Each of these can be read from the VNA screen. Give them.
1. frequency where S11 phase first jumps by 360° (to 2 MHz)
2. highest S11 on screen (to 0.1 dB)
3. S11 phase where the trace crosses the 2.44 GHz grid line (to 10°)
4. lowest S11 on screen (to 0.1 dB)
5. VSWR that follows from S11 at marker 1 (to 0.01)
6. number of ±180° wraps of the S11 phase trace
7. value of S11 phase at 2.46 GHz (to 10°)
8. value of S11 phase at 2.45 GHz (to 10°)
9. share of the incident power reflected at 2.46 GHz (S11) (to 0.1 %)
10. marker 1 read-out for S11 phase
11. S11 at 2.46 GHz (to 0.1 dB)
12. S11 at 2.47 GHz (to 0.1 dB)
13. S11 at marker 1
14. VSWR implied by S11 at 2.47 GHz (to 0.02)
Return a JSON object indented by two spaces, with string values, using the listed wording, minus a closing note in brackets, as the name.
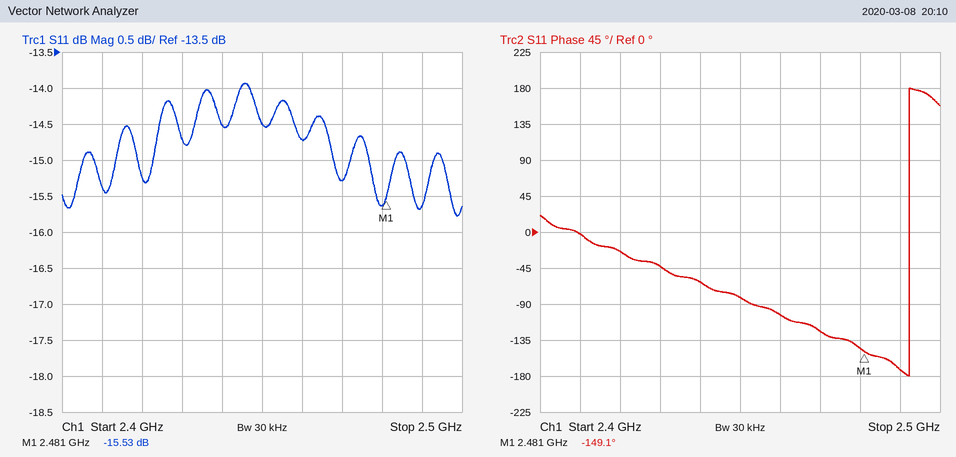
{
  "frequency where S11 phase first jumps by 360°": "2.492 GHz",
  "highest S11 on screen": "-13.9 dB",
  "S11 phase where the trace crosses the 2.44 GHz grid line": "-60°",
  "lowest S11 on screen": "-15.8 dB",
  "VSWR that follows from S11 at marker 1": "1.40",
  "number of ±180° wraps of the S11 phase trace": "1",
  "value of S11 phase at 2.46 GHz": "-100°",
  "value of S11 phase at 2.45 GHz": "-80°",
  "share of the incident power reflected at 2.46 GHz (S11)": "3.4 %",
  "marker 1 read-out for S11 phase": "-149.1°",
  "S11 at 2.46 GHz": "-14.7 dB",
  "S11 at 2.47 GHz": "-15.3 dB",
  "S11 at marker 1": "-15.53 dB",
  "VSWR implied by S11 at 2.47 GHz": "1.42"
}
